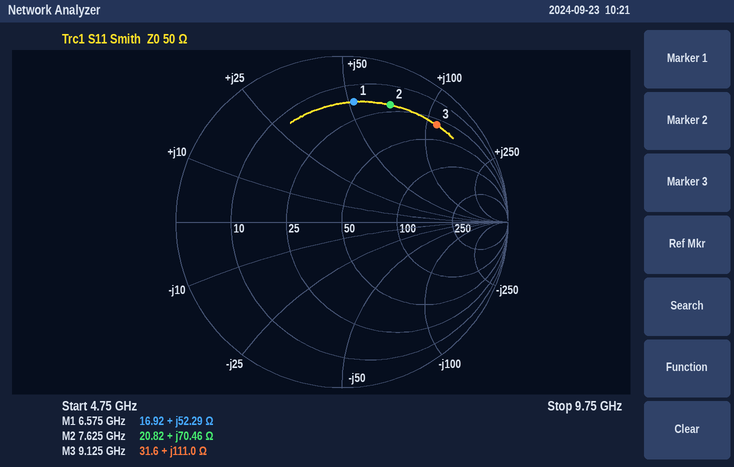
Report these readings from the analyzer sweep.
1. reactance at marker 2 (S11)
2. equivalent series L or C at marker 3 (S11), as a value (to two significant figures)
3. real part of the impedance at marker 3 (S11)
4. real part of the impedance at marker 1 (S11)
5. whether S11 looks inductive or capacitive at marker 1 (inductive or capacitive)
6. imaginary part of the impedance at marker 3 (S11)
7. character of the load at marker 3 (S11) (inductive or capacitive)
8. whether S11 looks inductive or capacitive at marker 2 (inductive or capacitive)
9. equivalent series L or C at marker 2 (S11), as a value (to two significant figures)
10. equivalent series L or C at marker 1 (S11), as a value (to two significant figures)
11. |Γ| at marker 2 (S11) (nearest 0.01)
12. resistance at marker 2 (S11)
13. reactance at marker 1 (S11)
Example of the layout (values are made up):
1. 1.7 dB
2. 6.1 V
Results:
1. +70.46 Ω
2. 1.9 nH
3. 31.6 Ω
4. 16.92 Ω
5. inductive
6. +111.0 Ω
7. inductive
8. inductive
9. 1.5 nH
10. 1.3 nH
11. 0.76
12. 20.82 Ω
13. +52.29 Ω
